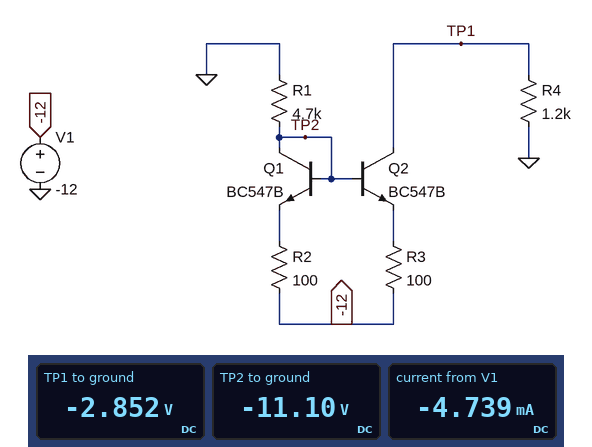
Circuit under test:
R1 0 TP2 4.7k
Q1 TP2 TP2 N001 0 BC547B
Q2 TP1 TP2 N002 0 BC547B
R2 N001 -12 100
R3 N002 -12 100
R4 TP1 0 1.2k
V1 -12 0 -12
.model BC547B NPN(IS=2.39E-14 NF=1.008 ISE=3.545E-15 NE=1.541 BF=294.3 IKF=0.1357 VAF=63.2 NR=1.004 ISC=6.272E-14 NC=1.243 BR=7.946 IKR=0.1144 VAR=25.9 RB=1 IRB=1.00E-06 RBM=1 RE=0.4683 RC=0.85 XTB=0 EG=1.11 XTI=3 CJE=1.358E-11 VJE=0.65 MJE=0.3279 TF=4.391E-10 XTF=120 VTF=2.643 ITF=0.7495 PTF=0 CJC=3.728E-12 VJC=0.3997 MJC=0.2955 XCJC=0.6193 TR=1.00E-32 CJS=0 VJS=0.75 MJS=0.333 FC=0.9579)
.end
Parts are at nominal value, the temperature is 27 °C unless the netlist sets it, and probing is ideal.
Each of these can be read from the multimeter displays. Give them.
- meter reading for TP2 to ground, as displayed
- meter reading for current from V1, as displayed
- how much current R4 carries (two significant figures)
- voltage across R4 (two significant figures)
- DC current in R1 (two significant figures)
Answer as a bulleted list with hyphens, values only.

- -11.10 V
- -4.739 mA
- 2.4 mA
- 2.9 V
- 2.4 mA
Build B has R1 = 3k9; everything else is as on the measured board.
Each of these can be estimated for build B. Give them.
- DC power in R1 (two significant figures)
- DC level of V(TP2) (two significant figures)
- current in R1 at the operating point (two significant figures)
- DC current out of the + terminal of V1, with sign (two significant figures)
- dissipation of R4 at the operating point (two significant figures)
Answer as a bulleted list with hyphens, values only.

- 31 mW
- -11 V
- 2.8 mA
- -5.7 mA
- 9.7 mW
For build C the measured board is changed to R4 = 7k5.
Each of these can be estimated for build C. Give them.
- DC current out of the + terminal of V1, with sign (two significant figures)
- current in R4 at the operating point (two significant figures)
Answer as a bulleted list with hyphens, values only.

- -3.9 mA
- 1.6 mA
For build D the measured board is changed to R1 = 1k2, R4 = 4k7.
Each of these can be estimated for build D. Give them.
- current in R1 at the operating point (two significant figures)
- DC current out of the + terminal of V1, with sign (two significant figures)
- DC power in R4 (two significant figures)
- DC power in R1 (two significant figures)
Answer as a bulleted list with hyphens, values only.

- 8.9 mA
- -11 mA
- 28 mW
- 96 mW
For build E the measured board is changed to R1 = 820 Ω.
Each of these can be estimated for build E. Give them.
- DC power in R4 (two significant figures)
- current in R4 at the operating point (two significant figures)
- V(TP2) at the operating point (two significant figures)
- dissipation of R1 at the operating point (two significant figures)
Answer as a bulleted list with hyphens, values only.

- 99 mW
- 9.1 mA
- -10 V
- 130 mW
